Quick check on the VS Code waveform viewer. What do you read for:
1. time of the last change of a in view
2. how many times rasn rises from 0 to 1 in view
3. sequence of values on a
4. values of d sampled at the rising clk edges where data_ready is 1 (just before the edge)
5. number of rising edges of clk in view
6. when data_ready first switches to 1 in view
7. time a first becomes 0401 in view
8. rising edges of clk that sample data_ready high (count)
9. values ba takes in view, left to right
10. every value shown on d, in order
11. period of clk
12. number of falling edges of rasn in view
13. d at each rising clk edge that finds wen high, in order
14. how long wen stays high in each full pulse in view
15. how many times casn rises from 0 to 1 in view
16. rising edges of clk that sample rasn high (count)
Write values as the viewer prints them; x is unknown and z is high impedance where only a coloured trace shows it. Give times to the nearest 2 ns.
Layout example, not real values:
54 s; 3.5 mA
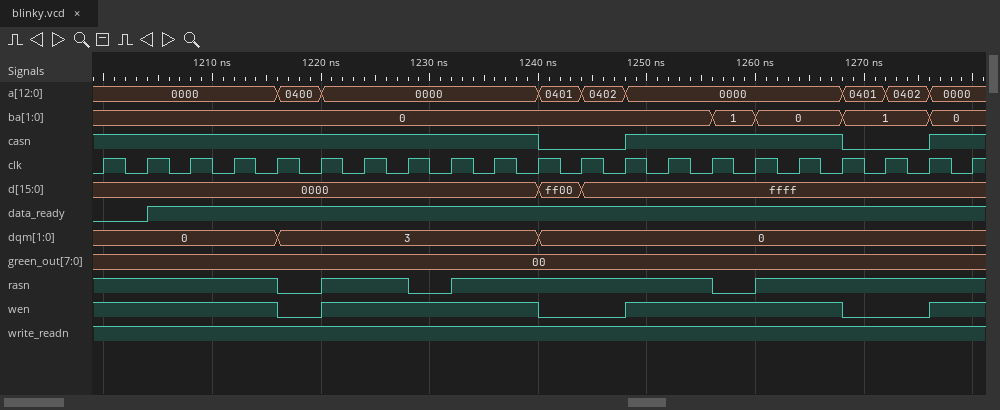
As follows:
1276 ns; 3; 0000, 0400, 0000, 0401, 0402, 0000, 0401, 0402, 0000; 0000, 0000, 0000, 0000, 0000, 0000, 0000, 0000, 0000, ff00, ffff, ffff, ffff, ffff, ffff, ffff, ffff, ffff, ffff; 21; 1204 ns; 1240 ns; 19; 0, 1, 0, 1, 0; 0000, ff00, ffff; 4 ns; 3; 0000, 0000, 0000, 0000, 0000, 0000, 0000, 0000, 0000, 0000, ffff, ffff, ffff, ffff, ffff, ffff; 20 ns, 20 ns; 2; 18
